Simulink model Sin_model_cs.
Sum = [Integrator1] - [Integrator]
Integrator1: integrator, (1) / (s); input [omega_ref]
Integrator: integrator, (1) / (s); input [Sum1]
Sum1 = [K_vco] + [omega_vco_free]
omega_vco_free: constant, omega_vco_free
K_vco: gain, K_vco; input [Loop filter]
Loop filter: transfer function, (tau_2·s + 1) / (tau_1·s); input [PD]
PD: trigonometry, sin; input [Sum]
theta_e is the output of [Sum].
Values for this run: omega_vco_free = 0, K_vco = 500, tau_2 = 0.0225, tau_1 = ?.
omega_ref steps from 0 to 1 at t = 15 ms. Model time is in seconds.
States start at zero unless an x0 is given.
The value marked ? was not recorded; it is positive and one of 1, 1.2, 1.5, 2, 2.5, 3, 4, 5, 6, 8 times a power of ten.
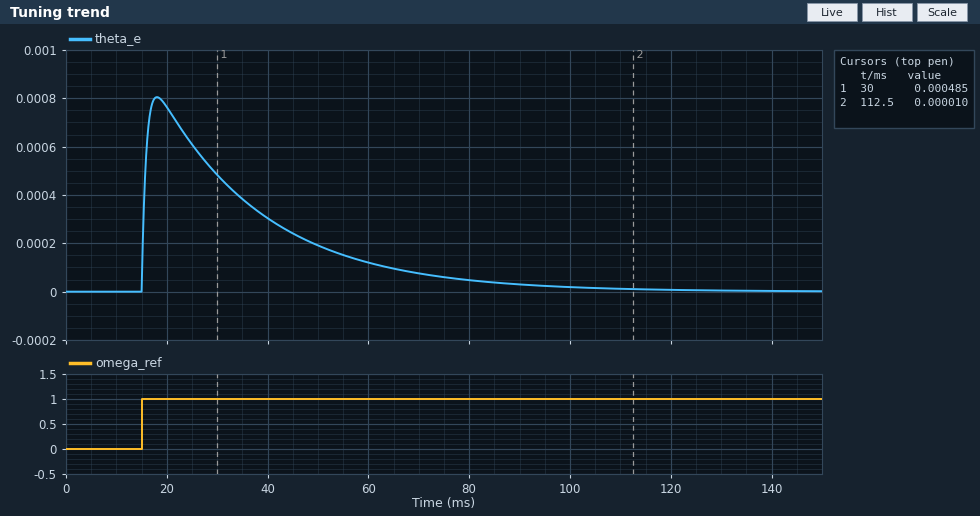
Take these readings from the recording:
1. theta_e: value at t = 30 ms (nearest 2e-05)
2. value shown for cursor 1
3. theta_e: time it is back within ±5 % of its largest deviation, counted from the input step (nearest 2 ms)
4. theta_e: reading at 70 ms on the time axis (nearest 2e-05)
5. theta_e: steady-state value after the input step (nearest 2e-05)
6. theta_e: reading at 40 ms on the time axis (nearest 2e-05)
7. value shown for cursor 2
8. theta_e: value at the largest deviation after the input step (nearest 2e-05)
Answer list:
0.00048
0.000485
68 ms
0.00008
0.00000
0.00030
0.000010
0.00080
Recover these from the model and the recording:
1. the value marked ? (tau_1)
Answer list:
0.01
